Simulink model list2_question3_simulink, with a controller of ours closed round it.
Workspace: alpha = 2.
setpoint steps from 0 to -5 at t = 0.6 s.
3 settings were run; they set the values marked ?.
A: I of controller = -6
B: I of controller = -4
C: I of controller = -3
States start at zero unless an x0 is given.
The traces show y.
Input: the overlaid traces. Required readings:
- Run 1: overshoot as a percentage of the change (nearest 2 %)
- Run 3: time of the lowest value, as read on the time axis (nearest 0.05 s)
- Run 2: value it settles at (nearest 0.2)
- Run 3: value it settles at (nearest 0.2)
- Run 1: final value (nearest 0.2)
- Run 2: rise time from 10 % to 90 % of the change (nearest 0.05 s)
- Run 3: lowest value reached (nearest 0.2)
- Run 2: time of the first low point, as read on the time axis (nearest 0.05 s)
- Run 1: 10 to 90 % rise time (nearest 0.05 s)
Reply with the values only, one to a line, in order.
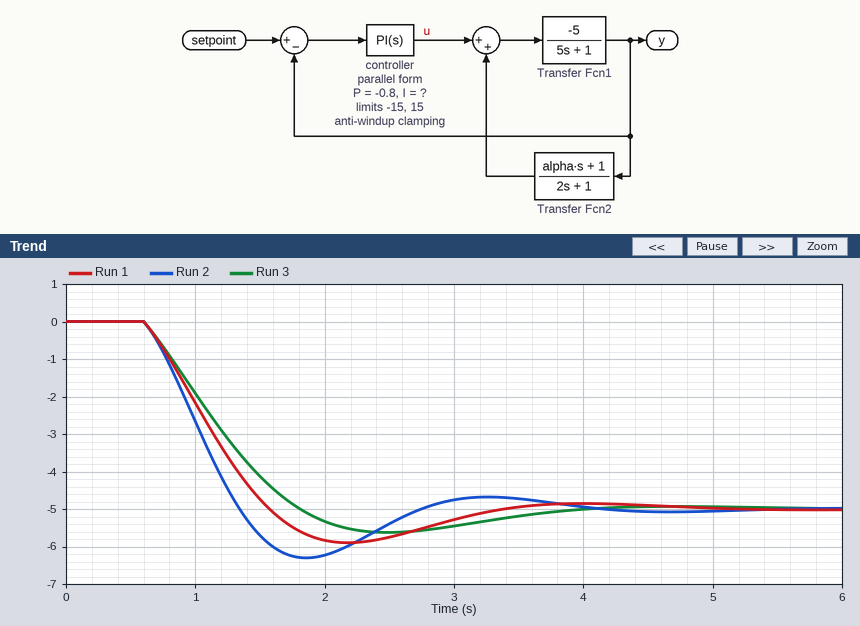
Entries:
18 %
2.50 s
-5.0
-5.0
-5.0
0.55 s
-5.6
1.85 s
0.75 s
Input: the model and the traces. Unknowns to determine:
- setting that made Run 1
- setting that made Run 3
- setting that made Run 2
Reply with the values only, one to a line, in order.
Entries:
B
C
A
